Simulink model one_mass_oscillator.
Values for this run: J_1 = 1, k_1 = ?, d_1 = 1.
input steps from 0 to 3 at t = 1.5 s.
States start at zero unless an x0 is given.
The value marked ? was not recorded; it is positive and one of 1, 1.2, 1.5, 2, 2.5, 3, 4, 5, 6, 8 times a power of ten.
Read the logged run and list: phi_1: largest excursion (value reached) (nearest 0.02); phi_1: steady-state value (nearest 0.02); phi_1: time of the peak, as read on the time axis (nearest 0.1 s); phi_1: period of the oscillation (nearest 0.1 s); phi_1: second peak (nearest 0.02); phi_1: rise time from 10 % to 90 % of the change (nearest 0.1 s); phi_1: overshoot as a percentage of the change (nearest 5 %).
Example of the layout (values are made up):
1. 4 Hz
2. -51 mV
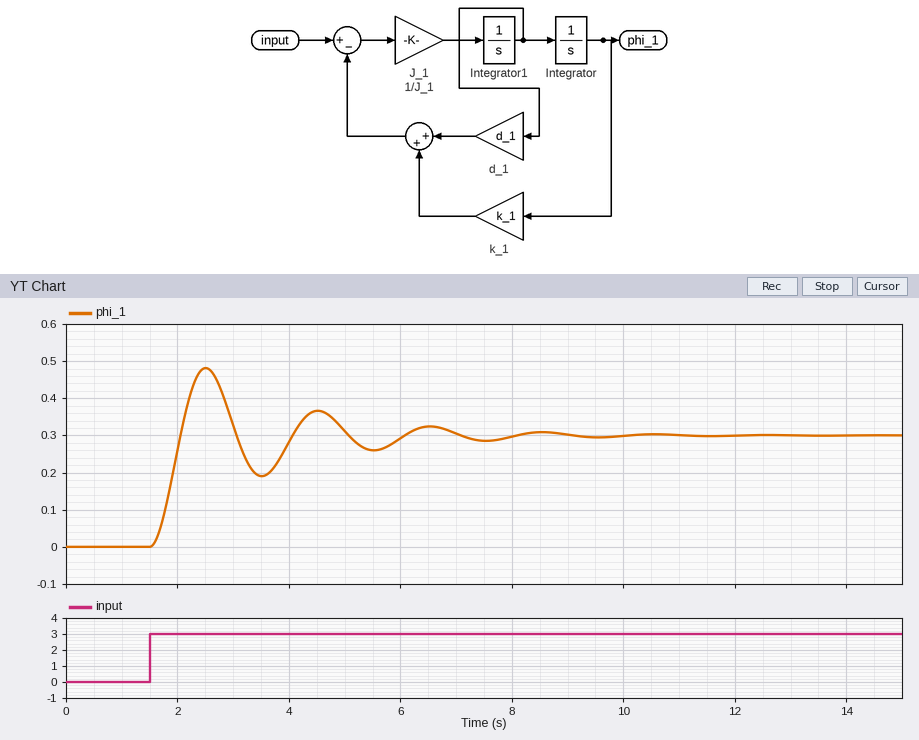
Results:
1. 0.48
2. 0.30
3. 2.5 s
4. 2.0 s
5. 0.36
6. 0.4 s
7. 60 %
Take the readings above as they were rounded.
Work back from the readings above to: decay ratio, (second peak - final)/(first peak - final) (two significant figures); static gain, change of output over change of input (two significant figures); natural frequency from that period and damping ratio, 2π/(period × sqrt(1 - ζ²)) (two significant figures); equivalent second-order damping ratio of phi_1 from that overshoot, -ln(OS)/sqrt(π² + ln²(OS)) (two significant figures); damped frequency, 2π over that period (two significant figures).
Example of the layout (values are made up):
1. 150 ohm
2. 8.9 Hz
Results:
1. 0.33
2. 0.10
3. 3.2 rad/s
4. 0.16
5. 3.1 rad/s
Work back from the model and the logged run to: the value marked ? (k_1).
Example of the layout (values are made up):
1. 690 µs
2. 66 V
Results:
1. 10
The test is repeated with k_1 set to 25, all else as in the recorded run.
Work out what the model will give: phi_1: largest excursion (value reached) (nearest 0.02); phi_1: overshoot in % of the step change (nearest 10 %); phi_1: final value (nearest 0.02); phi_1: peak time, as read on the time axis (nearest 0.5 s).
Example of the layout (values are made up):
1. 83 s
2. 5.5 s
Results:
1. 0.20
2. 70 %
3. 0.12
4. 2.0 s
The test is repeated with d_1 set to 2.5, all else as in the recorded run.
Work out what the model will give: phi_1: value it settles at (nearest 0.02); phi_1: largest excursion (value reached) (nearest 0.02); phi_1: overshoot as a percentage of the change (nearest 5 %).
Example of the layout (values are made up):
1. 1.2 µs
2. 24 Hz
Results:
1. 0.30
2. 0.38
3. 25 %
